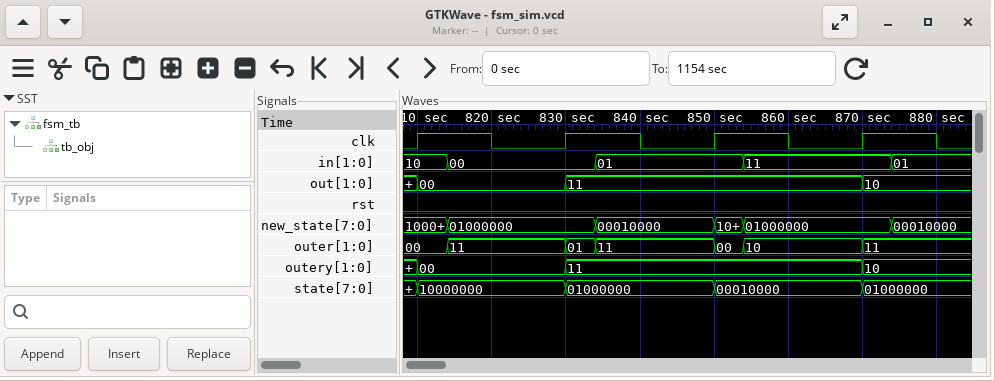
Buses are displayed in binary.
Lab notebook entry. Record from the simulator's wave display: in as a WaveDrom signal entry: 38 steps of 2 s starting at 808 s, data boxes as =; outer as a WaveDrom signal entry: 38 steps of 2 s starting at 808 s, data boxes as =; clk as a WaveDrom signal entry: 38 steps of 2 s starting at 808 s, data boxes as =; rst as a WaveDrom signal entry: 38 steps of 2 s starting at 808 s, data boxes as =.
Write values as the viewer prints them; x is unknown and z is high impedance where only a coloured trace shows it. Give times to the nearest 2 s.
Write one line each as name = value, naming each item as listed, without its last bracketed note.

in as a WaveDrom signal entry: 38 steps of 2 s starting at 808 s, data boxes as = = {name: 'in', wave: '=..=.........=.........=.........=....', data: '10 00 01 11 01'}
outer as a WaveDrom signal entry: 38 steps of 2 s starting at 808 s, data boxes as = = {name: 'outer', wave: '=..=.......=.=.......=.=.......=......', data: '00 11 01 11 00 10 11'}
clk as a WaveDrom signal entry: 38 steps of 2 s starting at 808 s, data boxes as = = {name: 'clk', wave: '01....0....1....0....1....0....1....0.'}
rst as a WaveDrom signal entry: 38 steps of 2 s starting at 808 s, data boxes as = = {name: 'rst', wave: '0.....................................'}
